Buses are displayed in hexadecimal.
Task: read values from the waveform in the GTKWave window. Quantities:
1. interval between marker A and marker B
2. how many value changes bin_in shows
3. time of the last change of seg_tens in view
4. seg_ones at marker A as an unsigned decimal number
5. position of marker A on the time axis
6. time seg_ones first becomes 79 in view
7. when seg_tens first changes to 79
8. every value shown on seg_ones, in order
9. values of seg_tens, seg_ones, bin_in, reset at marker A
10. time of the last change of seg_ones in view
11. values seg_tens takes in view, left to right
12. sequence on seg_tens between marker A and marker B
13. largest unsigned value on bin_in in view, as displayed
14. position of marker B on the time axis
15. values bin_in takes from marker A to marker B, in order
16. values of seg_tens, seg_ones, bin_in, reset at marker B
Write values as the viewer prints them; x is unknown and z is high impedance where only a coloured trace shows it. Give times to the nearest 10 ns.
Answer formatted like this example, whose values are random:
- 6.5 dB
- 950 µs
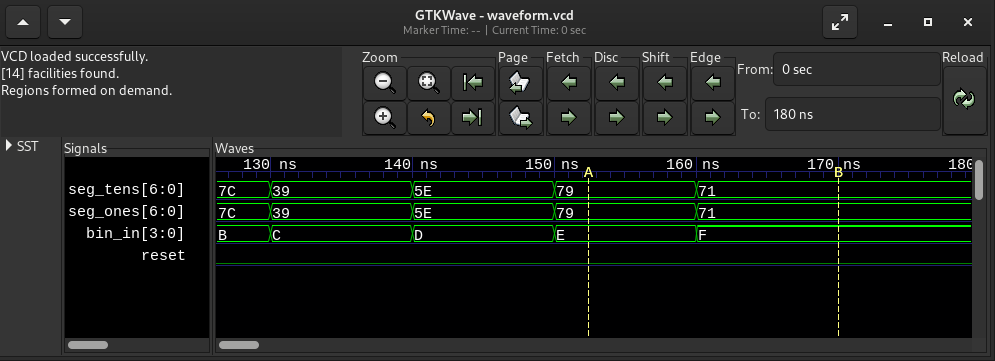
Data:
- 20 ns
- 4
- 160 ns
- 121
- 150 ns
- 150 ns
- 150 ns
- 7C, 39, 5E, 79, 71
- seg_tens=79, seg_ones=79, bin_in=E, reset=0
- 160 ns
- 7C, 39, 5E, 79, 71
- 79, 71
- F
- 170 ns
- E, F
- seg_tens=71, seg_ones=71, bin_in=F, reset=0
